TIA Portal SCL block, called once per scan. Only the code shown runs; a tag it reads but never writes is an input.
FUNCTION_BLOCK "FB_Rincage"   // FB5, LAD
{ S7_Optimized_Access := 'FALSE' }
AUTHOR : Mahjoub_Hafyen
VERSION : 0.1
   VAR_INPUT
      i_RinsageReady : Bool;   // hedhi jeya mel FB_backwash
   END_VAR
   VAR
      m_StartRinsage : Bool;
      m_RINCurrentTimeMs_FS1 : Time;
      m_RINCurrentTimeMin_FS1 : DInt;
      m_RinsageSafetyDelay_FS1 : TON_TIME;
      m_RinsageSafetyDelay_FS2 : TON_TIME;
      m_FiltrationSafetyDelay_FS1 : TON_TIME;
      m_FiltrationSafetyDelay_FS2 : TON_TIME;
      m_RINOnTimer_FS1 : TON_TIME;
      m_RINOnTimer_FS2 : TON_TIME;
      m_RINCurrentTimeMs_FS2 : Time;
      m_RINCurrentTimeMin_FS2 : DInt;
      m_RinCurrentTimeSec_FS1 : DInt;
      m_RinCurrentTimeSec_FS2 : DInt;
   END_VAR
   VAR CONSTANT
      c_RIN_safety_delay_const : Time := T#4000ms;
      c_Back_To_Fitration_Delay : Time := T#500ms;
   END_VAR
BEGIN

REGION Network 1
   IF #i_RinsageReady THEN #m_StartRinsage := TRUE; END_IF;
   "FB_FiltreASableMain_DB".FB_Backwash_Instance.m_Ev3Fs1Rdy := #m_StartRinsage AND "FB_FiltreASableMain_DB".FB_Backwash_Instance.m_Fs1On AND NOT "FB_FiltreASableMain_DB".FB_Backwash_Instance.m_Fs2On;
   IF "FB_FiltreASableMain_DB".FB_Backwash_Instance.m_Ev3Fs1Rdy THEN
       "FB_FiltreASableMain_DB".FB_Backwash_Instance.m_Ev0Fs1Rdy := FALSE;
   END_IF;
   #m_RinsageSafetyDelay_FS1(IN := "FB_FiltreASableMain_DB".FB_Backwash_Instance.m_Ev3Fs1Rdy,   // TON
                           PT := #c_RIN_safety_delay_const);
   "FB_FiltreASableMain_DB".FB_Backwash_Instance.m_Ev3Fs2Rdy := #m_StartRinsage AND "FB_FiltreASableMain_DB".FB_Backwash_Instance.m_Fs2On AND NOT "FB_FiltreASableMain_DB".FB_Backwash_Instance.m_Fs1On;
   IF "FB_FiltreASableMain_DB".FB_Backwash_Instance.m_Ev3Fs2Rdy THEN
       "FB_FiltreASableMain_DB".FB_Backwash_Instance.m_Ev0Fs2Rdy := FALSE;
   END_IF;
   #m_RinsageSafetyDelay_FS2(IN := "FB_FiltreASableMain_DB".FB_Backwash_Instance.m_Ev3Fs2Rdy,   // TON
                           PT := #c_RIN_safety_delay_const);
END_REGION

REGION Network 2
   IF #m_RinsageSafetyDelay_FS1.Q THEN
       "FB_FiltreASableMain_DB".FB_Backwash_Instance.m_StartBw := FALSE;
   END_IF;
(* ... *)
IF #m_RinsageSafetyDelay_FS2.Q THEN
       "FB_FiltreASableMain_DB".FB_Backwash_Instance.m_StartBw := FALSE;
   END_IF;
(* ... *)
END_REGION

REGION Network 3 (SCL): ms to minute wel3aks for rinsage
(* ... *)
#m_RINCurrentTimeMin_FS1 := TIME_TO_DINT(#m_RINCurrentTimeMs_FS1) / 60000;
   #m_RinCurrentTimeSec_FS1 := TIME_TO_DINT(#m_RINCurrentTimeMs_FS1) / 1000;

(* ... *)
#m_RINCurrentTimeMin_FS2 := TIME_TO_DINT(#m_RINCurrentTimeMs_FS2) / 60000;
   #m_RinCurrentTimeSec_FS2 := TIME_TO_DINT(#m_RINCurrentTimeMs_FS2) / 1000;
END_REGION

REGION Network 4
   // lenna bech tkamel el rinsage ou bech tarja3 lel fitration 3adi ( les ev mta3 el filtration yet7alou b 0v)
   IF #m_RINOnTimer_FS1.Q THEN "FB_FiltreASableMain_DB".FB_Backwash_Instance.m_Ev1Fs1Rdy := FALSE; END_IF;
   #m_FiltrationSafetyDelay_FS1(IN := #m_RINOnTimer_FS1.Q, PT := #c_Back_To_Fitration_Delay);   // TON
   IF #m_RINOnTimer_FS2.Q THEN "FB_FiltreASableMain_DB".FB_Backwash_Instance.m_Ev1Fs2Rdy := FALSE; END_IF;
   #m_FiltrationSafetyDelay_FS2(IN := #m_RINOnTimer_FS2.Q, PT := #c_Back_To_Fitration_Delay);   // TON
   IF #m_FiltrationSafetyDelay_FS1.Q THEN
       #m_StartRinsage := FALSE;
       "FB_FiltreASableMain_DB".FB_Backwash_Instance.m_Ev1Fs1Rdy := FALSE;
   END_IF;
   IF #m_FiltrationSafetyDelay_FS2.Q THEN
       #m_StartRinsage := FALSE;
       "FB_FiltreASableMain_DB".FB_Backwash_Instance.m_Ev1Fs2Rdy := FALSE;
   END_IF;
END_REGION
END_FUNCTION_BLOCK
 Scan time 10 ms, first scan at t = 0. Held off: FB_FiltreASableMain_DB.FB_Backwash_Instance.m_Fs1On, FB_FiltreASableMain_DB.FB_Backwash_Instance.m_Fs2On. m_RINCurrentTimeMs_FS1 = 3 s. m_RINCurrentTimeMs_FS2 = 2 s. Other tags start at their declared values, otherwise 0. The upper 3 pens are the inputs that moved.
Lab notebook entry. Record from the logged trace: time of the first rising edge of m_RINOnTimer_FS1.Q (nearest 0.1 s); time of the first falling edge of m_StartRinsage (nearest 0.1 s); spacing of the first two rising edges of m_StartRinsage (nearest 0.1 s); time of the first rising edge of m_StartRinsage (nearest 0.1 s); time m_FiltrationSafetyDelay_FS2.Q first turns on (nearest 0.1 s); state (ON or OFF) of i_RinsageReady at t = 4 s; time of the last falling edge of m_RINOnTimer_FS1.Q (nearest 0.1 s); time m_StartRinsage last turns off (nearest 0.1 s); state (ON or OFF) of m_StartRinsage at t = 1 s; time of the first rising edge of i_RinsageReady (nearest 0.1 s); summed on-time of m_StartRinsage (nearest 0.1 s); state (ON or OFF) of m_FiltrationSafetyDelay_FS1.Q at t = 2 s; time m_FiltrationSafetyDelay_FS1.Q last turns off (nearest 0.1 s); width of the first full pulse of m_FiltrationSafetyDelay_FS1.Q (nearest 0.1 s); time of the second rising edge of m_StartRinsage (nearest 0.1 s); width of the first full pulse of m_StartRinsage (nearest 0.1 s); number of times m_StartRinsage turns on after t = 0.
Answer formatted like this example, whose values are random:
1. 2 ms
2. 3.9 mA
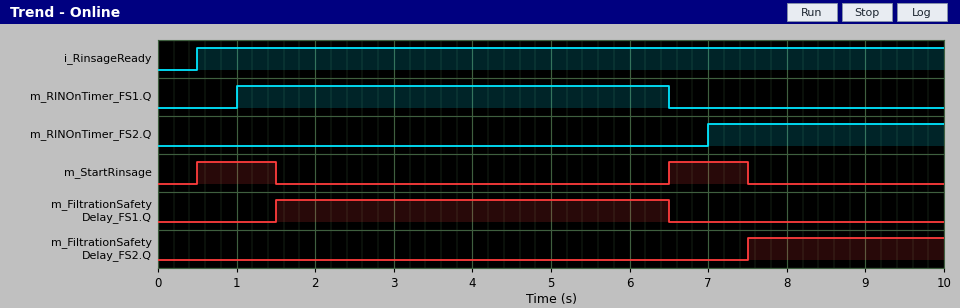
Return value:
1. 1.0 s
2. 1.5 s
3. 6.0 s
4. 0.5 s
5. 7.5 s
6. ON
7. 6.5 s
8. 7.5 s
9. ON
10. 0.5 s
11. 2.0 s
12. ON
13. 6.5 s
14. 5.0 s
15. 6.5 s
16. 1.0 s
17. 2
